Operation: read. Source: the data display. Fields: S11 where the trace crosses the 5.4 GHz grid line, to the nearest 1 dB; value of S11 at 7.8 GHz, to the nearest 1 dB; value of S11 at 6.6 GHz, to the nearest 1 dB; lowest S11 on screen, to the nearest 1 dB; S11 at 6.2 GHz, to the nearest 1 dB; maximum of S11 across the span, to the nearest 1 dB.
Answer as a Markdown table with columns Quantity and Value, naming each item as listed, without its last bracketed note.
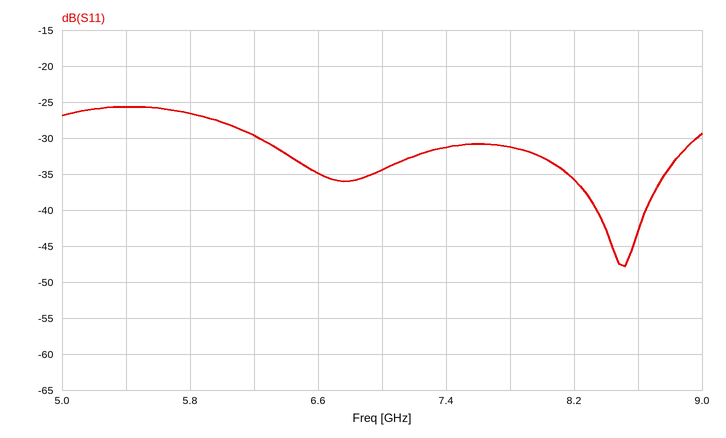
| Quantity | Value |
|---|---|
| S11 where the trace crosses the 5.4 GHz grid line, to the nearest 1 dB | -26 dB |
| value of S11 at 7.8 GHz, to the nearest 1 dB | -31 dB |
| value of S11 at 6.6 GHz, to the nearest 1 dB | -35 dB |
| lowest S11 on screen, to the nearest 1 dB | -48 dB |
| S11 at 6.2 GHz, to the nearest 1 dB | -30 dB |
| maximum of S11 across the span, to the nearest 1 dB | -26 dB |
